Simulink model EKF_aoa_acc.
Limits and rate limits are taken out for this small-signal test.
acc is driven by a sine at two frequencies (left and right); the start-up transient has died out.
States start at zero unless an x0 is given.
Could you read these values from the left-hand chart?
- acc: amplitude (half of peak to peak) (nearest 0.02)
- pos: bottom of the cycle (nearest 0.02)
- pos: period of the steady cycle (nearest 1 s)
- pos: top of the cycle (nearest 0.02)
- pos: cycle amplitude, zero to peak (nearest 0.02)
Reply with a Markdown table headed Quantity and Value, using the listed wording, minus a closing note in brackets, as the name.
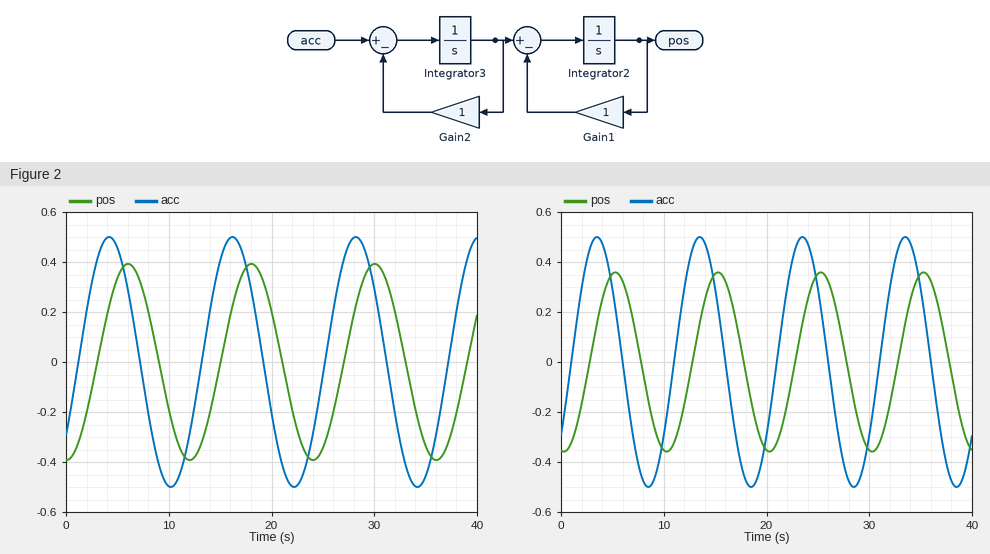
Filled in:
| Quantity | Value |
|---|---|
| acc: amplitude (half of peak to peak) | 0.50 |
| pos: bottom of the cycle | -0.40 |
| pos: period of the steady cycle | 12 s |
| pos: top of the cycle | 0.40 |
| pos: cycle amplitude, zero to peak | 0.40 |
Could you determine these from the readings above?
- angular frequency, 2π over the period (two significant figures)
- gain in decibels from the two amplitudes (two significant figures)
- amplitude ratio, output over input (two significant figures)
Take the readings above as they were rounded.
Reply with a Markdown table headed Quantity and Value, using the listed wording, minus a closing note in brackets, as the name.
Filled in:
| Quantity | Value |
|---|---|
| angular frequency, 2π over the period | 0.52 rad/s |
| gain in decibels from the two amplitudes | -1.9 dB |
| amplitude ratio, output over input | 0.80 |
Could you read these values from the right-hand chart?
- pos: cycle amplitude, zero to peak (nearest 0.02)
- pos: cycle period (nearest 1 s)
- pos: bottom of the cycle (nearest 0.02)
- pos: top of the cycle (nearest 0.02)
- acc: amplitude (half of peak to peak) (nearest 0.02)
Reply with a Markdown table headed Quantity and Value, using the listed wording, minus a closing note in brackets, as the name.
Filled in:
| Quantity | Value |
|---|---|
| pos: cycle amplitude, zero to peak | 0.36 |
| pos: cycle period | 10 s |
| pos: bottom of the cycle | -0.36 |
| pos: top of the cycle | 0.36 |
| acc: amplitude (half of peak to peak) | 0.50 |
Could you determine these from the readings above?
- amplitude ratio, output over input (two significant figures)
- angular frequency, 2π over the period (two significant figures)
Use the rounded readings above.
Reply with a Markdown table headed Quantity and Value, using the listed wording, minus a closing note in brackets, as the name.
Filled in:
| Quantity | Value |
|---|---|
| amplitude ratio, output over input | 0.72 |
| angular frequency, 2π over the period | 0.63 rad/s |
